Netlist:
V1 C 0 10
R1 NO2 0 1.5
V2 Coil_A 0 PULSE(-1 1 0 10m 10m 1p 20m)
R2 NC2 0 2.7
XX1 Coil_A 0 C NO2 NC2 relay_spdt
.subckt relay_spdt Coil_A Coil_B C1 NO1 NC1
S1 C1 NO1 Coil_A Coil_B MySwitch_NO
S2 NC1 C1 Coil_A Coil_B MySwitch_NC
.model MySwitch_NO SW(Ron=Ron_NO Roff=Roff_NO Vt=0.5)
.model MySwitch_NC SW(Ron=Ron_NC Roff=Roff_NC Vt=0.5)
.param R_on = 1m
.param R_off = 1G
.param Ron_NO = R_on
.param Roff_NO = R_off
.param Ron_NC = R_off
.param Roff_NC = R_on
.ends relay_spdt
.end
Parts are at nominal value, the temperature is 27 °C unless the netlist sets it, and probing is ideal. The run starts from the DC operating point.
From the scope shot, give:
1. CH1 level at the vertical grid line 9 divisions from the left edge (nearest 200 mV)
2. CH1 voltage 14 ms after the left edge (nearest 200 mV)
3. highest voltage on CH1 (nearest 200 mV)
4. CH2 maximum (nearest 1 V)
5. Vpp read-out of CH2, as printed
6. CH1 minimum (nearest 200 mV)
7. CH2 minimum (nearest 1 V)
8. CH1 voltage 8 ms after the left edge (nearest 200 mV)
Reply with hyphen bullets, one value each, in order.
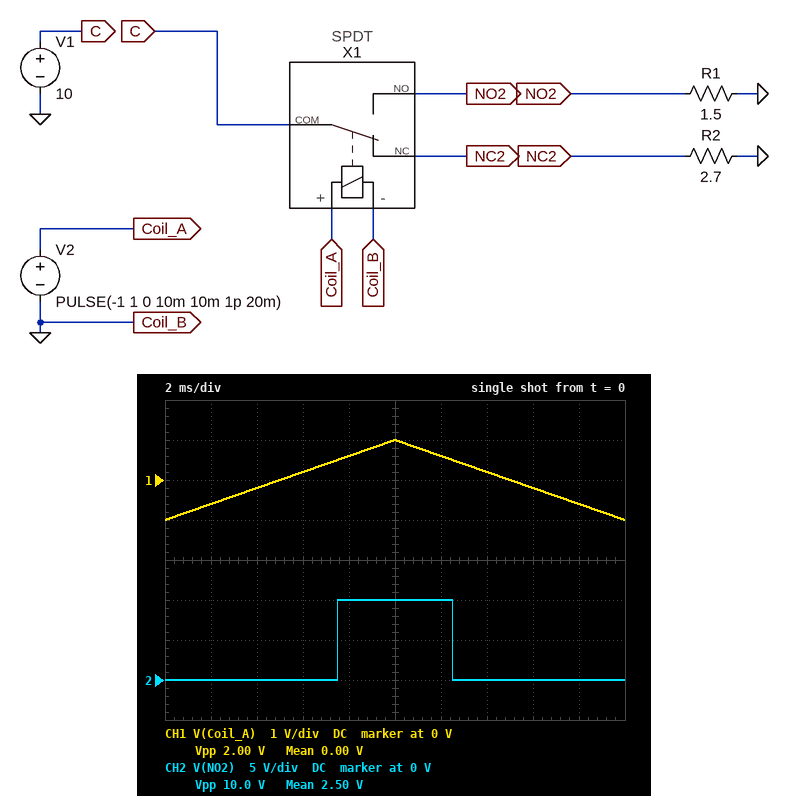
- -600 mV
- 200 mV
- 1.0 V
- 10 V
- 10.0 V
- -1.0 V
- 0 V
- 600 mV
